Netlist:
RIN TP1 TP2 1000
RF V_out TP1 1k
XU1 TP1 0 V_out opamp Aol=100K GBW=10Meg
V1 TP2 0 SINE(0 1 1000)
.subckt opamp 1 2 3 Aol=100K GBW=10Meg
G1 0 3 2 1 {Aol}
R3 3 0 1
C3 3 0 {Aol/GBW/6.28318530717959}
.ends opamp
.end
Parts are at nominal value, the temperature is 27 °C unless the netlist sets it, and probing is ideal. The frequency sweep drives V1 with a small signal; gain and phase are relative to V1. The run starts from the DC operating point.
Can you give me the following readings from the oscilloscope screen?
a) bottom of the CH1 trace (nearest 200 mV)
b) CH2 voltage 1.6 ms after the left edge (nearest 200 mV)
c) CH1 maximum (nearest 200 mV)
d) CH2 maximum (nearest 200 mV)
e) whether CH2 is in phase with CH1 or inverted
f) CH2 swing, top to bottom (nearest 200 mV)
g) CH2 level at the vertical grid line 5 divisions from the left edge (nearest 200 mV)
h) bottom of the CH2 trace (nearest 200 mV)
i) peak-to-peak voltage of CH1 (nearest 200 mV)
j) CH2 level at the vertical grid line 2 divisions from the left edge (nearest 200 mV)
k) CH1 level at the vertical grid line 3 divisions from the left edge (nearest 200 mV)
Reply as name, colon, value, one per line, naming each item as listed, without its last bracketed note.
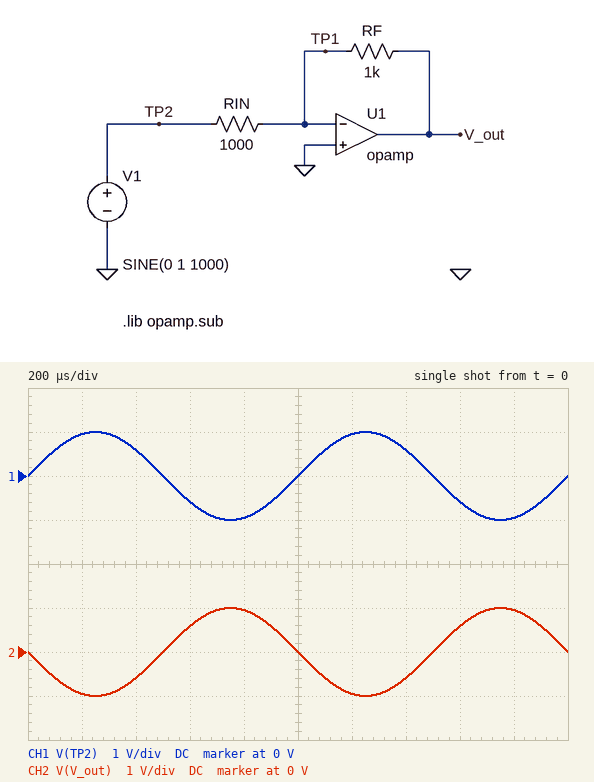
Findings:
bottom of the CH1 trace: -1.0 V
CH2 voltage 1.6 ms after the left edge: 600 mV
CH1 maximum: 1.0 V
CH2 maximum: 1.0 V
whether CH2 is in phase with CH1 or inverted: inverted
CH2 swing, top to bottom: 2.0 V
CH2 level at the vertical grid line 5 divisions from the left edge: 0 V
bottom of the CH2 trace: -1.0 V
peak-to-peak voltage of CH1: 2.0 V
CH2 level at the vertical grid line 2 divisions from the left edge: -600 mV
CH1 level at the vertical grid line 3 divisions from the left edge: -600 mV
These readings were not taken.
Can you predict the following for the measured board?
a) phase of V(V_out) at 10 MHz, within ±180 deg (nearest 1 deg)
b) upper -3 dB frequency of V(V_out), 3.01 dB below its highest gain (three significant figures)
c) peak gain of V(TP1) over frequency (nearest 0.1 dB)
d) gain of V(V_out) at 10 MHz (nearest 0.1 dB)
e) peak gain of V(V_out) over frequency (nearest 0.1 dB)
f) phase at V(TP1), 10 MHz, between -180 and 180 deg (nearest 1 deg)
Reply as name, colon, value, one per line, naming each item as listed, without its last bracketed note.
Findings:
phase of V(V_out) at 10 MHz, within ±180 deg: 117 deg
upper -3 dB frequency of V(V_out), 3.01 dB below its highest gain: 5.00 MHz
peak gain of V(TP1) over frequency: -6.0 dB
gain of V(V_out) at 10 MHz: -7.0 dB
peak gain of V(V_out) over frequency: 0 dB
phase at V(TP1), 10 MHz, between -180 and 180 deg: 27 deg
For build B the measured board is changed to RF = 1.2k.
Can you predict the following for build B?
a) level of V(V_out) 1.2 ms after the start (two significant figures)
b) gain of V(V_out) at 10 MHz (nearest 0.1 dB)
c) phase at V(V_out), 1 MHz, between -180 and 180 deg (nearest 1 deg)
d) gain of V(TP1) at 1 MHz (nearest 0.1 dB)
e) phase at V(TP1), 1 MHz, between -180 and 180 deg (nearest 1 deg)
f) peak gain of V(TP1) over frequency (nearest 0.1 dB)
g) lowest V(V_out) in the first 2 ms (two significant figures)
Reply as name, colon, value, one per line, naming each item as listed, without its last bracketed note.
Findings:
level of V(V_out) 1.2 ms after the start: -1.1 V
gain of V(V_out) at 10 MHz: -6.1 dB
phase at V(V_out), 1 MHz, between -180 and 180 deg: 168 deg
gain of V(TP1) at 1 MHz: -18.6 dB
phase at V(TP1), 1 MHz, between -180 and 180 deg: 78 deg
peak gain of V(TP1) over frequency: -5.3 dB
lowest V(V_out) in the first 2 ms: -1.2 V
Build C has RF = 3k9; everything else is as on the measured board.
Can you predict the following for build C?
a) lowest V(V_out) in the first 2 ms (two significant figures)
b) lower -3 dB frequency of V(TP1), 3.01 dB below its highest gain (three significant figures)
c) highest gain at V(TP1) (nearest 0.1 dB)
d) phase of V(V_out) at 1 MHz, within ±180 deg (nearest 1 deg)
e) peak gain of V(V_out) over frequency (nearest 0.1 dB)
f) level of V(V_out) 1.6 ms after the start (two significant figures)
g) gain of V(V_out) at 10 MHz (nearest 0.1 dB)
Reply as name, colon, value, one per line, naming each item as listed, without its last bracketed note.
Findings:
lowest V(V_out) in the first 2 ms: -3.9 V
lower -3 dB frequency of V(TP1), 3.01 dB below its highest gain: 2.04 MHz
highest gain at V(TP1): -2.0 dB
phase of V(V_out) at 1 MHz, within ±180 deg: 154 deg
peak gain of V(V_out) over frequency: 11.8 dB
level of V(V_out) 1.6 ms after the start: 2.3 V
gain of V(V_out) at 10 MHz: -2.2 dB
